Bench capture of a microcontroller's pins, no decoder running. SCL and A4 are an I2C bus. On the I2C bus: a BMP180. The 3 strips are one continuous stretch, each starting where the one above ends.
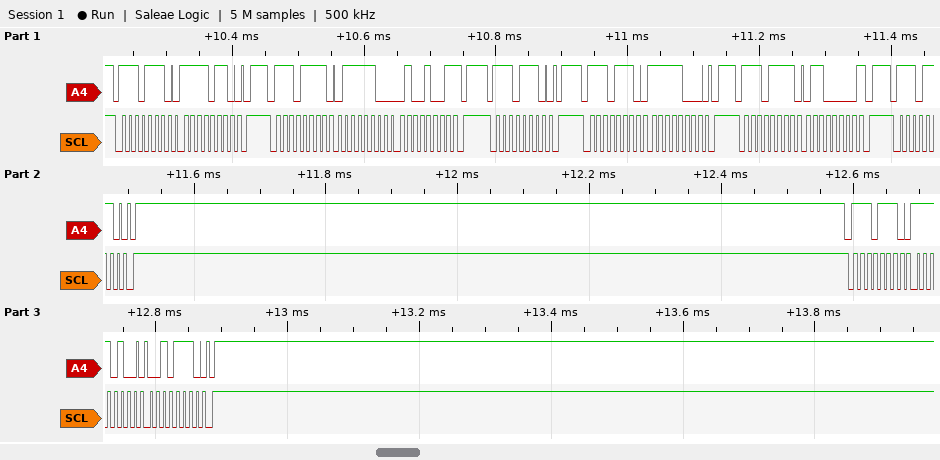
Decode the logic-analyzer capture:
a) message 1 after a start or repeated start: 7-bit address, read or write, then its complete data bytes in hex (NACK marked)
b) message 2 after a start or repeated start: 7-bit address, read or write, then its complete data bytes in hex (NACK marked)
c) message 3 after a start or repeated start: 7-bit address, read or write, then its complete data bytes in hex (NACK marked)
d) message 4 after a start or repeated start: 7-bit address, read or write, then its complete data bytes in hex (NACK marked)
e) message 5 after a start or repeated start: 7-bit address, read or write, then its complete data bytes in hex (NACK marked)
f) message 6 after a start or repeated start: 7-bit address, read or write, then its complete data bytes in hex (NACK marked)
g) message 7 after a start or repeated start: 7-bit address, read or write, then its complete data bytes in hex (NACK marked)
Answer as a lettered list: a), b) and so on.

a) 0x77 write: F6
b) 0x77 read: 7C 49 NACK
c) 0x77 write
d) 0x77 write: F8
e) 0x77 read: 60 NACK
f) 0x77 write
g) 0x77 write: F4 2E
